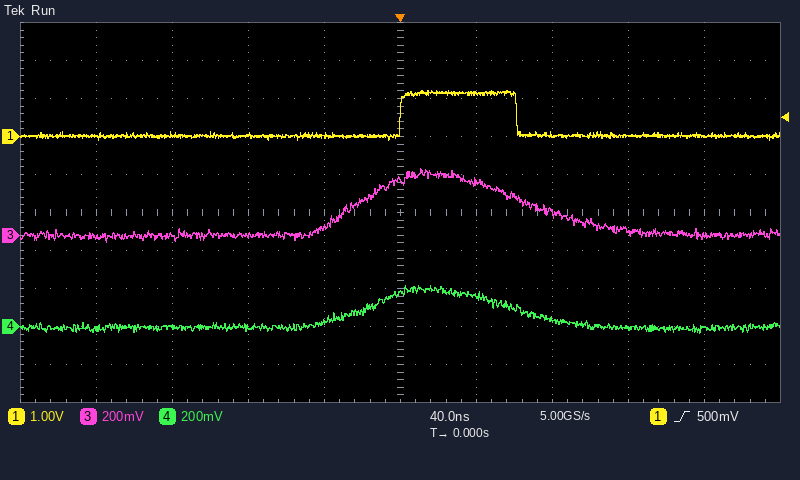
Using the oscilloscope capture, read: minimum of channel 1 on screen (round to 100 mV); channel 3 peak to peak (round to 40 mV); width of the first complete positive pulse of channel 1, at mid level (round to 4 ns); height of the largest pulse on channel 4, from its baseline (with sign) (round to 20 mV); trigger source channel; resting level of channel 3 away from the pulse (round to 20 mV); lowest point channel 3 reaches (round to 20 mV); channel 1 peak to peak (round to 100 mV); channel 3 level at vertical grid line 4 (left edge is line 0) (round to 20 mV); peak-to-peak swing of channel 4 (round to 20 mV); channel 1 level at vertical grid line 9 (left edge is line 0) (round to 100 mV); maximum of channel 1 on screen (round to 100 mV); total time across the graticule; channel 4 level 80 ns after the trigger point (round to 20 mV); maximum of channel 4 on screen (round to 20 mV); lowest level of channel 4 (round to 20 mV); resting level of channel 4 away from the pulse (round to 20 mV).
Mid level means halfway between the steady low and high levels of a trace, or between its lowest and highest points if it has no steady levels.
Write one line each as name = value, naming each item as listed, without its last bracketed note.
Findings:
minimum of channel 1 on screen = -100 mV
channel 3 peak to peak = 400 mV
width of the first complete positive pulse of channel 1, at mid level = 60 ns
height of the largest pulse on channel 4, from its baseline (with sign) = +220 mV
trigger source channel = channel 1
resting level of channel 3 away from the pulse = 0 mV
lowest point channel 3 reaches = -40 mV
channel 1 peak to peak = 1.3 V
channel 3 level at vertical grid line 4 (left edge is line 0) = 40 mV
peak-to-peak swing of channel 4 = 260 mV
channel 1 level at vertical grid line 9 (left edge is line 0) = 0.0 V
maximum of channel 1 on screen = 1.2 V
total time across the graticule = 400 ns
channel 4 level 80 ns after the trigger point = 40 mV
maximum of channel 4 on screen = 220 mV
lowest level of channel 4 = -40 mV
resting level of channel 4 away from the pulse = 0 mV
